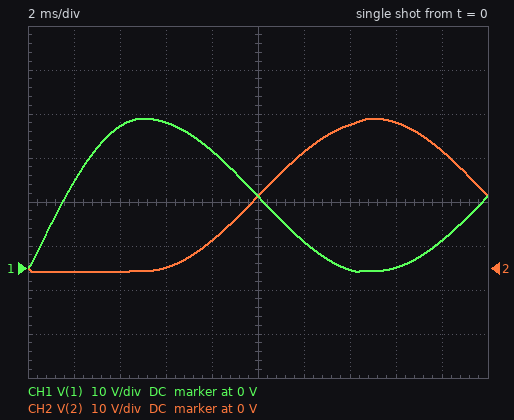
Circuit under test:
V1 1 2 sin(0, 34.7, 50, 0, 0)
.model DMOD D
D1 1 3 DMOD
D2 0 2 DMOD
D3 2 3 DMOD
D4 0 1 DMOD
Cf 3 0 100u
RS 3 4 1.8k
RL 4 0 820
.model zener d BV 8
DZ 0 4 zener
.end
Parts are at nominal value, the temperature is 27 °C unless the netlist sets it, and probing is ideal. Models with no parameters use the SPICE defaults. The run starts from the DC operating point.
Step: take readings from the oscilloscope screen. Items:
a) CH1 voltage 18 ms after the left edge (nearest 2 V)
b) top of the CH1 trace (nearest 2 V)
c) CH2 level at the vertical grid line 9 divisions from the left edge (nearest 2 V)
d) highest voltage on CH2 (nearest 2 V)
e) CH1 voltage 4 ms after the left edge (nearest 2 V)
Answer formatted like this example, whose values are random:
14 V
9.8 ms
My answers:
6 V
34 V
26 V
34 V
32 V
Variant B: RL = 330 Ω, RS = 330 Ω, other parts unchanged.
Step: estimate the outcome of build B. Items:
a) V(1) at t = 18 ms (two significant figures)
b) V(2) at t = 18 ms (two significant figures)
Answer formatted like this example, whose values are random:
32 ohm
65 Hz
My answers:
5.4 V
26 V
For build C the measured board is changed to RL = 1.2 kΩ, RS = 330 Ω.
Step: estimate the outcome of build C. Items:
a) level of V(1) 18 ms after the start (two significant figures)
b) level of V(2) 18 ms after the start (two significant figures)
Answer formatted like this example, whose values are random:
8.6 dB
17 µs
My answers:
5.4 V
26 V
